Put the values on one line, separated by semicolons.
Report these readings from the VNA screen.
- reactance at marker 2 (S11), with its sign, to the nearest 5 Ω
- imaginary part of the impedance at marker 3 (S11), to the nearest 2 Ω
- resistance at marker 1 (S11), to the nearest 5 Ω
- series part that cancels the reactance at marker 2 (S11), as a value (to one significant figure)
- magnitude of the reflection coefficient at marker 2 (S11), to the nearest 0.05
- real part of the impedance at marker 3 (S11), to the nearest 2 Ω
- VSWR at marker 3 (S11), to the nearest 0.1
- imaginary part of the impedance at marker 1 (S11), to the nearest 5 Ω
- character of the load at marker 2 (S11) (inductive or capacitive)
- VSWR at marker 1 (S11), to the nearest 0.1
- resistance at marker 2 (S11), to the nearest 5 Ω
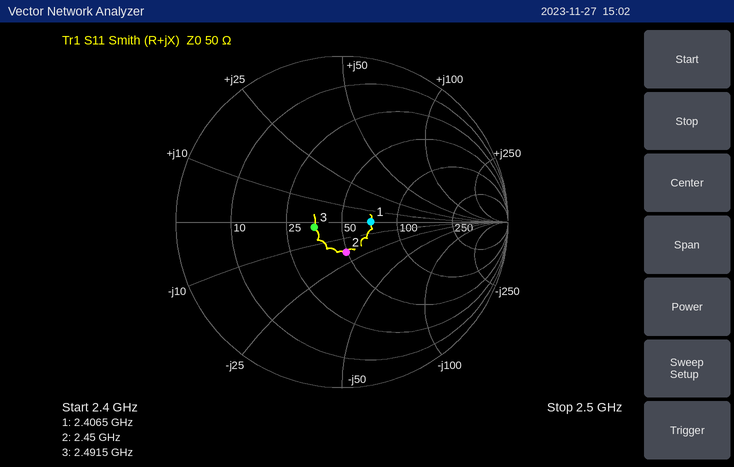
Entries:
-20 Ω; -2 Ω; 70 Ω; 1 nH; 0.20; 36 Ω; 1.4; 0 Ω; capacitive; 1.4; 50 Ω
